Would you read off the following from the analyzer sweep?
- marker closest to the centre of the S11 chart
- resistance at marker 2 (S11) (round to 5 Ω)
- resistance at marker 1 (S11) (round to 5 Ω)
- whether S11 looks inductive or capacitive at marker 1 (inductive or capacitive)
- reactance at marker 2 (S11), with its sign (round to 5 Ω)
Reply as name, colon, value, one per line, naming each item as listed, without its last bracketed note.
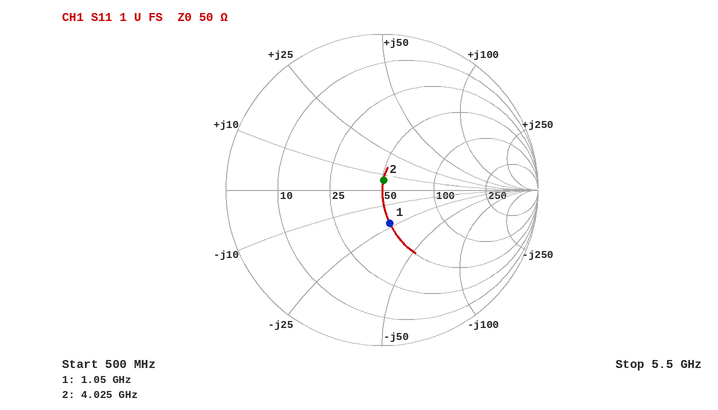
marker closest to the centre of the S11 chart: marker 2
resistance at marker 2 (S11): 50 Ω
resistance at marker 1 (S11): 50 Ω
whether S11 looks inductive or capacitive at marker 1: capacitive
reactance at marker 2 (S11), with its sign: +5 Ω
